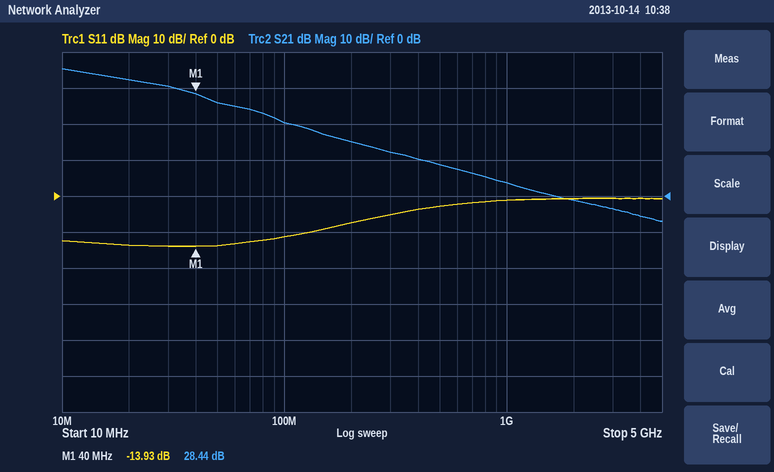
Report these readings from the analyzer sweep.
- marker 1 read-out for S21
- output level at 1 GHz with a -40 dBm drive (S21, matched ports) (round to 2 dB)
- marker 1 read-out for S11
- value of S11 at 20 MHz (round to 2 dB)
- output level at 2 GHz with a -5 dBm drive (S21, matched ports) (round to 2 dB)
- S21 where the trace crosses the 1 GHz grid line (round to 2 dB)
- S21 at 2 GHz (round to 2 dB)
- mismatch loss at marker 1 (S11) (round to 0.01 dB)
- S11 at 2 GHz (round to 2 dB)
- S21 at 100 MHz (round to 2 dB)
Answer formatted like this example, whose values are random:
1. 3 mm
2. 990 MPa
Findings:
1. 28.44 dB
2. -36 dBm
3. -13.93 dB
4. -14 dB
5. -6 dBm
6. 4 dB
7. -2 dB
8. 0.18 dB
9. 0 dB
10. 20 dB
